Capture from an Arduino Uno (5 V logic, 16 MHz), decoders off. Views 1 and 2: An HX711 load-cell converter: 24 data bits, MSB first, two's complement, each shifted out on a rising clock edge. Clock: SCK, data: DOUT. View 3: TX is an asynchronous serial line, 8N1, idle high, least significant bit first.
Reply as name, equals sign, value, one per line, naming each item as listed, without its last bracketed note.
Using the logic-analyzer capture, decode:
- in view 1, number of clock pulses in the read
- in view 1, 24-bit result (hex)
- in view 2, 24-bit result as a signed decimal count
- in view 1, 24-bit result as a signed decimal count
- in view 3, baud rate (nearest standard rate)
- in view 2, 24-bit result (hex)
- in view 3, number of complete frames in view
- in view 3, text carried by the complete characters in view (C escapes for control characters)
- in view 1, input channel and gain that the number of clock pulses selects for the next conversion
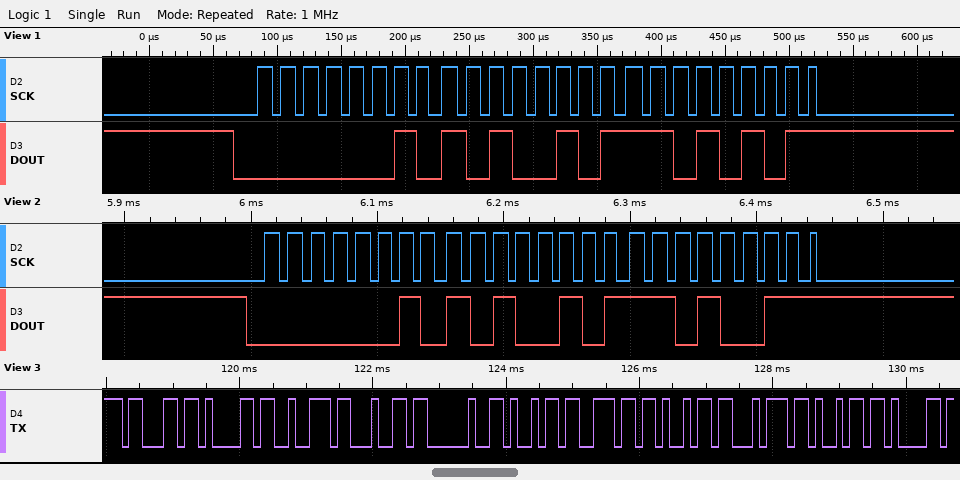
in view 1, number of clock pulses in the read = 25
in view 1, 24-bit result = 0x02A5D5
in view 2, 24-bit result as a signed decimal count = 173523
in view 1, 24-bit result as a signed decimal count = 173525
in view 3, baud rate = 9600 baud
in view 2, 24-bit result = 0x02A5D3
in view 3, number of complete frames in view = 11
in view 3, text carried by the complete characters in view = "card initia"
in view 1, input channel and gain that the number of clock pulses selects for the next conversion = channel A, gain 128
